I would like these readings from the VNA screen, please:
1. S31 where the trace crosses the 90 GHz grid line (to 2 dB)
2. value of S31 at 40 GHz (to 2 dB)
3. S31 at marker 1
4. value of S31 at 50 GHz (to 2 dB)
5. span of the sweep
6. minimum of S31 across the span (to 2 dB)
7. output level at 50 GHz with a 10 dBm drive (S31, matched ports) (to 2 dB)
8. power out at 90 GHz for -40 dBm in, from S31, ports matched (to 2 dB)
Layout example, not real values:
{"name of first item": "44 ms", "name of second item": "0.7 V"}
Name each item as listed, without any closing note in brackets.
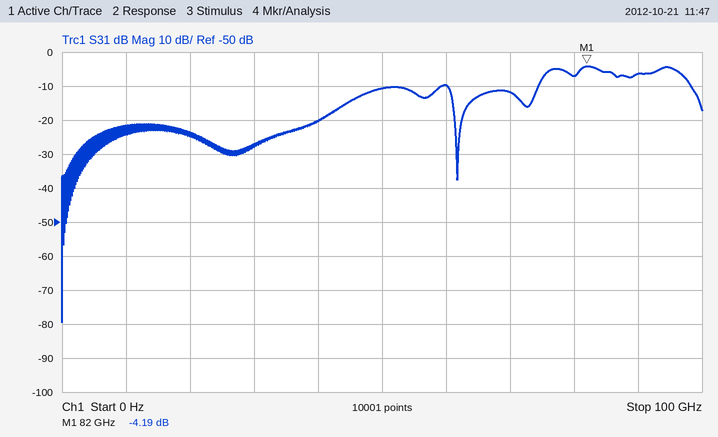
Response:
{"S31 where the trace crosses the 90 GHz grid line": "-6 dB", "value of S31 at 40 GHz": "-20 dB", "S31 at marker 1": "-4.19 dB", "value of S31 at 50 GHz": "-10 dB", "span of the sweep": "100 GHz", "minimum of S31 across the span": "-80 dB", "output level at 50 GHz with a 10 dBm drive (S31, matched ports)": "0 dBm", "power out at 90 GHz for -40 dBm in, from S31, ports matched": "-46 dBm"}
